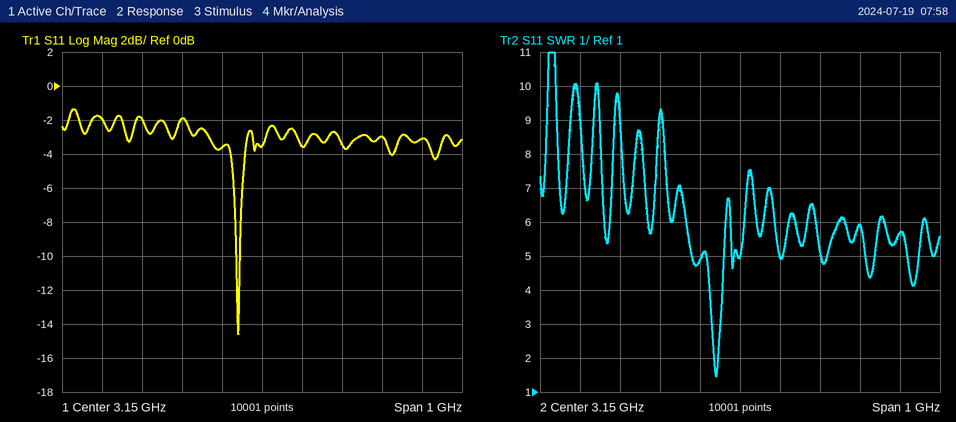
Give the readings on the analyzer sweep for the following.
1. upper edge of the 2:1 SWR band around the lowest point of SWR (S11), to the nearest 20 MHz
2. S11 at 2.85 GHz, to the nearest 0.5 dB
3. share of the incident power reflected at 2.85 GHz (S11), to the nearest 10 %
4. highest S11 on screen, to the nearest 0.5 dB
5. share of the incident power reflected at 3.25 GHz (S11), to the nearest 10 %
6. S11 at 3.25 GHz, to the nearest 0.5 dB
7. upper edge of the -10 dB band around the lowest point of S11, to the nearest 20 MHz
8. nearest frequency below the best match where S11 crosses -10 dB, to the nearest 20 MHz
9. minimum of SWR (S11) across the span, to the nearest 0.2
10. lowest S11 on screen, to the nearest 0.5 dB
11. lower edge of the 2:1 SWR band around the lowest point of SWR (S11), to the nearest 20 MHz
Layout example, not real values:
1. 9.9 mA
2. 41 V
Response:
1. 3.10 GHz
2. -2.0 dB
3. 60 %
4. -1.5 dB
5. 40 %
6. -3.5 dB
7. 3.10 GHz
8. 3.08 GHz
9. 1.4
10. -14.5 dB
11. 3.08 GHz
